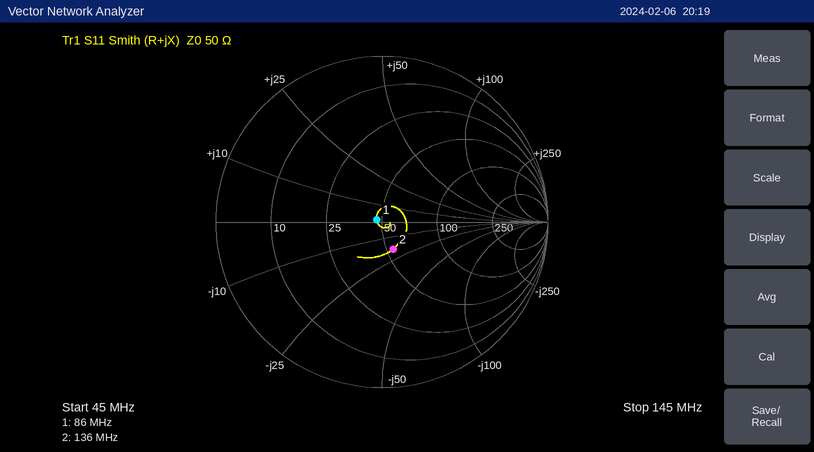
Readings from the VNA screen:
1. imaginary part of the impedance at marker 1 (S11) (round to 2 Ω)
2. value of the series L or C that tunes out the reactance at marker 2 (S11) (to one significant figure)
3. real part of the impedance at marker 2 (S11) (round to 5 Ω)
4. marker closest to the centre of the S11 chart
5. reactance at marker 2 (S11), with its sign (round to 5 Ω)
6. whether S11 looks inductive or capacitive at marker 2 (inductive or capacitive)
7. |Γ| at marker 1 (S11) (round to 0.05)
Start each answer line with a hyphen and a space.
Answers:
- +2 Ω
- 20 nH
- 55 Ω
- marker 1
- -20 Ω
- capacitive
- 0.05
